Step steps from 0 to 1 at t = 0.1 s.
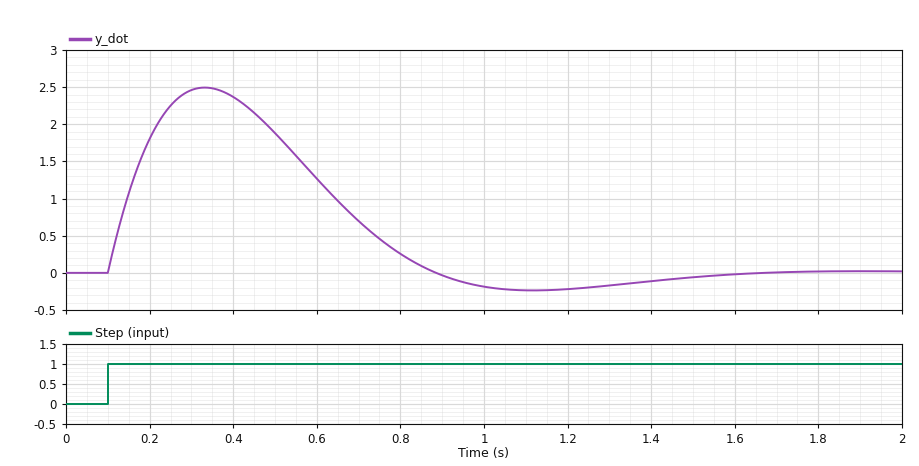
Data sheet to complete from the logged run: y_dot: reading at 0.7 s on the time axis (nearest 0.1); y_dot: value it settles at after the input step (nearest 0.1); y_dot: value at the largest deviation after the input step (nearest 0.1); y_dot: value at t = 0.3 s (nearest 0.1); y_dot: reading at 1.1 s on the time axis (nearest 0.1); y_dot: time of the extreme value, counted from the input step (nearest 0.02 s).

0.7
0.0
2.5
2.5
-0.2
0.24 s
